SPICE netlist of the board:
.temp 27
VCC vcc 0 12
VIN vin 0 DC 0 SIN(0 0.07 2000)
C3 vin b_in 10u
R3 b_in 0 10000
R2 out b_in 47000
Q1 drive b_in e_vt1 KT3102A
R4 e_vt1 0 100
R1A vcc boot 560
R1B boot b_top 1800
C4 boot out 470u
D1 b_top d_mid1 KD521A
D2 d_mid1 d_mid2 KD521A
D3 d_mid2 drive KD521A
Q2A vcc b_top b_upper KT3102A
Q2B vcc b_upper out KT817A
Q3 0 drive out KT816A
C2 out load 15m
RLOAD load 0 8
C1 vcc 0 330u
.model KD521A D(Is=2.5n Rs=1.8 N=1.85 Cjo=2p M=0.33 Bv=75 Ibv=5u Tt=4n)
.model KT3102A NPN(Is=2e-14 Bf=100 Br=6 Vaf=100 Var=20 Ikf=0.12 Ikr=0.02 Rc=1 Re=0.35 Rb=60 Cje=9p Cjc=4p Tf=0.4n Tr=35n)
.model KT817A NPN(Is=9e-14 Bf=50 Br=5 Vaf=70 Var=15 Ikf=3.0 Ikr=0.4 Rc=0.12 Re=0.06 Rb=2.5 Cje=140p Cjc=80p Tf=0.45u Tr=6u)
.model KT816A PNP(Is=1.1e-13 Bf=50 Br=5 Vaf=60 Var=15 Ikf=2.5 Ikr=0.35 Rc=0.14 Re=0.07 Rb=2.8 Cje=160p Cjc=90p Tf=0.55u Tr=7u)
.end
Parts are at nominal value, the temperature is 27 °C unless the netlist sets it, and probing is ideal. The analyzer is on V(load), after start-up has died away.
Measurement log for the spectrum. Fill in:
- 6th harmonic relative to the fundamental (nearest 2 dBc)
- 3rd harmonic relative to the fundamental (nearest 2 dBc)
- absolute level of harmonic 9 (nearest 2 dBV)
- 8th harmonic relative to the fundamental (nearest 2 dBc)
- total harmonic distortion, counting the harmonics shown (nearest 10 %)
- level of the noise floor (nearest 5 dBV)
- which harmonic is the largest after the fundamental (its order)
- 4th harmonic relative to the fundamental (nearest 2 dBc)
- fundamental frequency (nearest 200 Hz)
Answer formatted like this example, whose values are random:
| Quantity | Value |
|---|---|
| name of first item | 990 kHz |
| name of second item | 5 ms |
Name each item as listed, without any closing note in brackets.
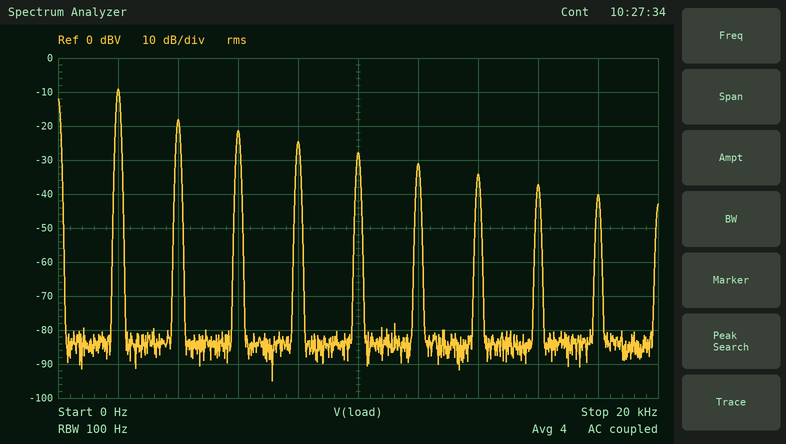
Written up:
| Quantity | Value |
|---|---|
| 6th harmonic relative to the fundamental | -22 dBc |
| 3rd harmonic relative to the fundamental | -12 dBc |
| absolute level of harmonic 9 | -40 dBV |
| 8th harmonic relative to the fundamental | -28 dBc |
| total harmonic distortion, counting the harmonics shown | 50 % |
| level of the noise floor | -85 dBV |
| which harmonic is the largest after the fundamental | 2 |
| 4th harmonic relative to the fundamental | -16 dBc |
| fundamental frequency | 2.0 kHz |
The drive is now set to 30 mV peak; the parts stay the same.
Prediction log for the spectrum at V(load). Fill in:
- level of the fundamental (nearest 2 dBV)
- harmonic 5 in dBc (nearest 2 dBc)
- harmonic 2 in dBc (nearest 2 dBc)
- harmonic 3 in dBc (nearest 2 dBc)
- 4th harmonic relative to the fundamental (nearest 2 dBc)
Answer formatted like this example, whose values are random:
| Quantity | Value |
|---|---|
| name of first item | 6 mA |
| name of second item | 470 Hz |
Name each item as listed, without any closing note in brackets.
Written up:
| Quantity | Value |
|---|---|
| level of the fundamental | -20 dBV |
| harmonic 5 in dBc | -56 dBc |
| harmonic 2 in dBc | -22 dBc |
| harmonic 3 in dBc | -34 dBc |
| 4th harmonic relative to the fundamental | -44 dBc |
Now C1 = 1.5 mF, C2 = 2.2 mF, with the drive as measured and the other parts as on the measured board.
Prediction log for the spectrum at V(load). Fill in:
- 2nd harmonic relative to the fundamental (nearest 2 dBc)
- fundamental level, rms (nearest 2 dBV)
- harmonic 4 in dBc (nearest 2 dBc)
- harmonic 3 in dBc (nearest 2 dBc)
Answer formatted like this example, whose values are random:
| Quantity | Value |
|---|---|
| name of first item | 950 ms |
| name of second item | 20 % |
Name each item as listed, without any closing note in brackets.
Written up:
| Quantity | Value |
|---|---|
| 2nd harmonic relative to the fundamental | -10 dBc |
| fundamental level, rms | -10 dBV |
| harmonic 4 in dBc | -18 dBc |
| harmonic 3 in dBc | -14 dBc |
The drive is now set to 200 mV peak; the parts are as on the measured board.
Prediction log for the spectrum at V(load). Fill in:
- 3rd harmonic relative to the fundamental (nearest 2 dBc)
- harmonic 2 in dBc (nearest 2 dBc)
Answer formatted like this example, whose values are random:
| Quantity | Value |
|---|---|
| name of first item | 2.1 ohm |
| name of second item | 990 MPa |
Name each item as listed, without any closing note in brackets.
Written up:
| Quantity | Value |
|---|---|
| 3rd harmonic relative to the fundamental | -8 dBc |
| harmonic 2 in dBc | -6 dBc |
